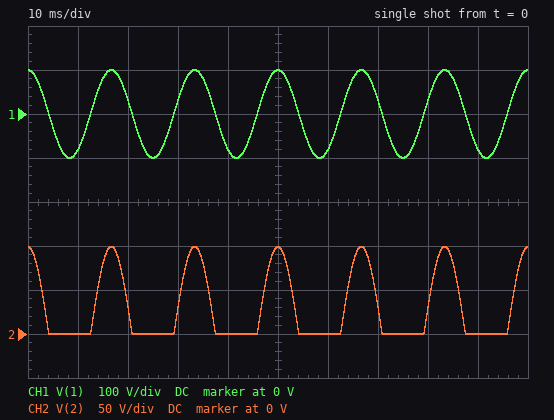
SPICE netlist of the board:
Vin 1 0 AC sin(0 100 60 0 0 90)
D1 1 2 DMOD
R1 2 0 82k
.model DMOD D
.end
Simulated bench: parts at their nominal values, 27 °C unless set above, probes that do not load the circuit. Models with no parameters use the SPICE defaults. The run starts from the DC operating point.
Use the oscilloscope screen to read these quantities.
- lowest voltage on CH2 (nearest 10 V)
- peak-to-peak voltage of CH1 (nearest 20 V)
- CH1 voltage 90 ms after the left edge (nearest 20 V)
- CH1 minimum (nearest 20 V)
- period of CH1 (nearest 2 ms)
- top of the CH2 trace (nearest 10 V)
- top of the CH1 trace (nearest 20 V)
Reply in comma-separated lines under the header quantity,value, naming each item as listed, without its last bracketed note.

quantity,value
lowest voltage on CH2,0 V
peak-to-peak voltage of CH1,200 V
CH1 voltage 90 ms after the left edge,-80 V
CH1 minimum,-100 V
period of CH1,16 ms
top of the CH2 trace,100 V
top of the CH1 trace,100 V
